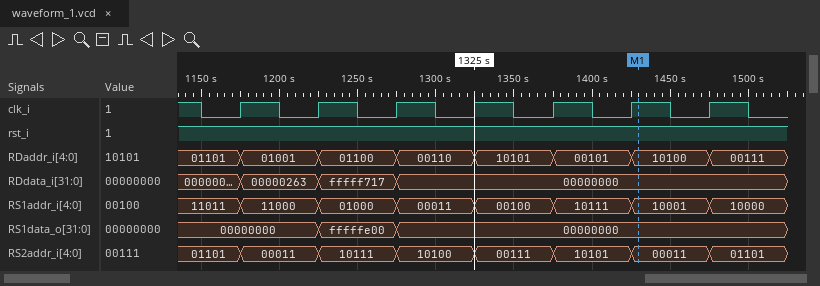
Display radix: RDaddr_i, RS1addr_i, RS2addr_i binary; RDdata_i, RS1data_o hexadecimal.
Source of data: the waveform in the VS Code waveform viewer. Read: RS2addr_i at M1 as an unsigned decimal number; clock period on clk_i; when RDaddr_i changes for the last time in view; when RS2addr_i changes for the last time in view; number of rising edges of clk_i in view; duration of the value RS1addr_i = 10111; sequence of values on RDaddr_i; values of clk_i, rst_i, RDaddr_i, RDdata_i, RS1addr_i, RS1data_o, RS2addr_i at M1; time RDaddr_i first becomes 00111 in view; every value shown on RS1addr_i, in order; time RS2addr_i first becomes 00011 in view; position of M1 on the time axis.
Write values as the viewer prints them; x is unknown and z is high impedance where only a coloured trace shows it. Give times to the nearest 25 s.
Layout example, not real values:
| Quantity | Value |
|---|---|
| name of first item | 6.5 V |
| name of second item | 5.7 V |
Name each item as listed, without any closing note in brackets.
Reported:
| Quantity | Value |
|---|---|
| RS2addr_i at M1 as an unsigned decimal number | 3 |
| clock period on clk_i | 50 s |
| when RDaddr_i changes for the last time in view | 1475 s |
| when RS2addr_i changes for the last time in view | 1475 s |
| number of rising edges of clk_i in view | 7 |
| duration of the value RS1addr_i = 10111 | 50 s |
| sequence of values on RDaddr_i | 01101, 01001, 01100, 00110, 10101, 00101, 10100, 00111 |
| values of clk_i, rst_i, RDaddr_i, RDdata_i, RS1addr_i, RS1data_o, RS2addr_i at M1 | clk_i=1, rst_i=1, RDaddr_i=10100, RDdata_i=00000000, RS1addr_i=10001, RS1data_o=00000000, RS2addr_i=00011 |
| time RDaddr_i first becomes 00111 in view | 1475 s |
| every value shown on RS1addr_i, in order | 11011, 11000, 01000, 00011, 00100, 10111, 10001, 10000 |
| time RS2addr_i first becomes 00011 in view | 1175 s |
| position of M1 on the time axis | 1425 s |
